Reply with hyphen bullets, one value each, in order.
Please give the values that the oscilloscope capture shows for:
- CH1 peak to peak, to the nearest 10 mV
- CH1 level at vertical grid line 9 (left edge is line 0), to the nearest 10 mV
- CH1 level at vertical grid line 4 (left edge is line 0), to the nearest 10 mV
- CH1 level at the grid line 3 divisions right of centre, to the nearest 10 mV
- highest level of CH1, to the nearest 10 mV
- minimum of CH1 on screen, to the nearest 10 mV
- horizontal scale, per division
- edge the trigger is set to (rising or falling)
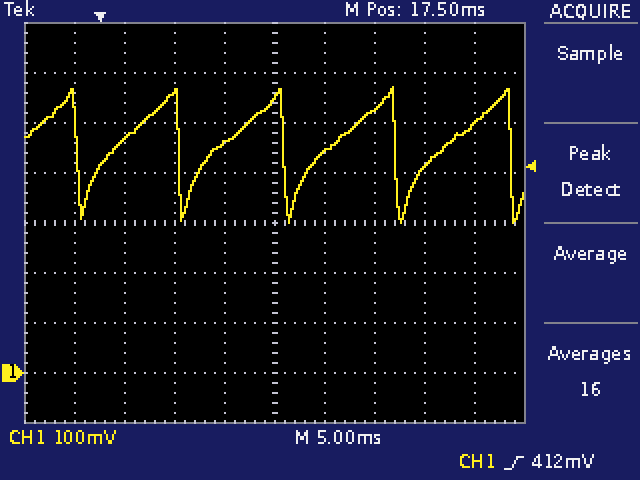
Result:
- 270 mV
- 500 mV
- 460 mV
- 410 mV
- 570 mV
- 300 mV
- 5 ms
- rising
